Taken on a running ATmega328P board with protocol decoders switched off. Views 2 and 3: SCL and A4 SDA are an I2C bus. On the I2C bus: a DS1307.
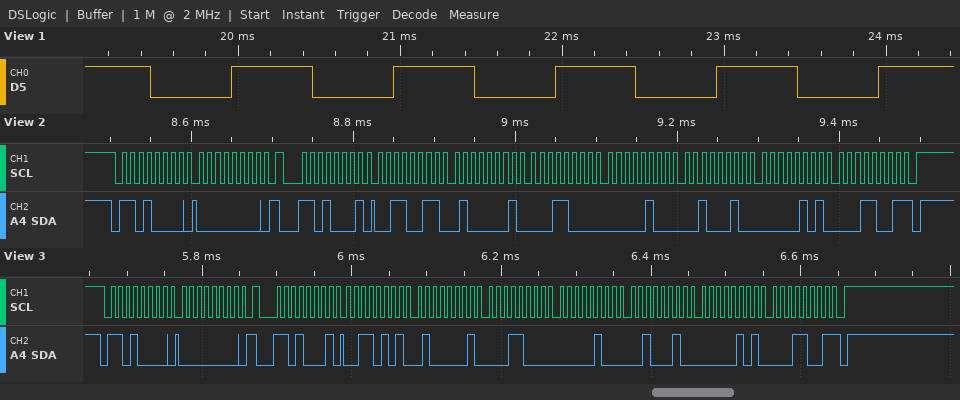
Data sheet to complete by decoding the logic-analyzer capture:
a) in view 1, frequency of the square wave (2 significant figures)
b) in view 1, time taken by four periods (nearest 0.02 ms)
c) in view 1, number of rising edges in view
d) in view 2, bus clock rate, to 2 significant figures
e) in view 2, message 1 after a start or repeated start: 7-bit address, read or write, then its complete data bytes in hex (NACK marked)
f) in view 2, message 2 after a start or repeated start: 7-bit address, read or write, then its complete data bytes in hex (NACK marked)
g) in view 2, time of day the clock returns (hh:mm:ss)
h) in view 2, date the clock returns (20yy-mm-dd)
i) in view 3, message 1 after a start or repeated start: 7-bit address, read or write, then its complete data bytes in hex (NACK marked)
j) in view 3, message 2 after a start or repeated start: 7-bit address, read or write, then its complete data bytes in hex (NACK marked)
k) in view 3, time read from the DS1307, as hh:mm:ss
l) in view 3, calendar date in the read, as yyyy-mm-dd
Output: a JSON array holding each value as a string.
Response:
["1.00 kHz", "4.00 ms", "5", "100 kHz", "0x68 write: 00", "0x68 read: 33 41 18 04 22 05 19 NACK", "18:41:33", "2019-05-22", "0x68 write: 00", "0x68 read: 35 41 18 04 22 05 19 NACK", "18:41:35", "2019-05-22"]
